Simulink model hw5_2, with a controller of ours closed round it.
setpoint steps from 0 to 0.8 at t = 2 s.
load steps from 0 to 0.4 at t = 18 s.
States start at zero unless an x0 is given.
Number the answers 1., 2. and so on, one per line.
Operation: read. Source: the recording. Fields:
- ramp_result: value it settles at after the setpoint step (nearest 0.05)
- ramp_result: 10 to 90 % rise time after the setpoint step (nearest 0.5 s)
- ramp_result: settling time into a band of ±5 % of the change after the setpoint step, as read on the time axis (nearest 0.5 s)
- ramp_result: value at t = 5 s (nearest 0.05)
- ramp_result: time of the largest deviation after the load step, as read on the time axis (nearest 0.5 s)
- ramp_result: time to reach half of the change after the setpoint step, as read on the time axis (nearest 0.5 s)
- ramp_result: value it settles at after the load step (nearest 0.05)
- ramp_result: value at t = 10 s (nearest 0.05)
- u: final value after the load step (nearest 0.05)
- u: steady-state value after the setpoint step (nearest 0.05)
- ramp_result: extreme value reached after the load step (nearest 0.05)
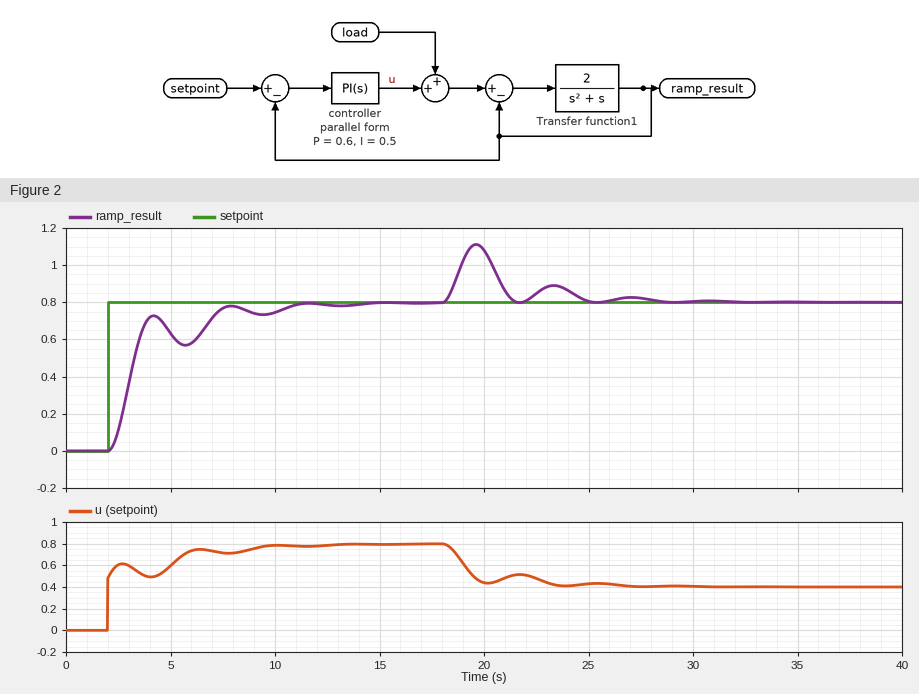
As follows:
1. 0.80
2. 1.5 s
3. 10.5 s
4. 0.65
5. 19.5 s
6. 3.0 s
7. 0.80
8. 0.75
9. 0.40
10. 0.80
11. 1.10
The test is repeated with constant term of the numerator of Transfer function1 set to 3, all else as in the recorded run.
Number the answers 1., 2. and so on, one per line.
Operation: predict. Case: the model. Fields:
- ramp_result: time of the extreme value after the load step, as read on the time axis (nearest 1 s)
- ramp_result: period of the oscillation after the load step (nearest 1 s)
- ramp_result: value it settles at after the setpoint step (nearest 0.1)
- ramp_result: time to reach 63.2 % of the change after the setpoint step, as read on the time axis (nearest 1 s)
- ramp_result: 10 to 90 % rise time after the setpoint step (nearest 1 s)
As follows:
1. 19 s
2. 3 s
3. 0.8
4. 3 s
5. 4 s
